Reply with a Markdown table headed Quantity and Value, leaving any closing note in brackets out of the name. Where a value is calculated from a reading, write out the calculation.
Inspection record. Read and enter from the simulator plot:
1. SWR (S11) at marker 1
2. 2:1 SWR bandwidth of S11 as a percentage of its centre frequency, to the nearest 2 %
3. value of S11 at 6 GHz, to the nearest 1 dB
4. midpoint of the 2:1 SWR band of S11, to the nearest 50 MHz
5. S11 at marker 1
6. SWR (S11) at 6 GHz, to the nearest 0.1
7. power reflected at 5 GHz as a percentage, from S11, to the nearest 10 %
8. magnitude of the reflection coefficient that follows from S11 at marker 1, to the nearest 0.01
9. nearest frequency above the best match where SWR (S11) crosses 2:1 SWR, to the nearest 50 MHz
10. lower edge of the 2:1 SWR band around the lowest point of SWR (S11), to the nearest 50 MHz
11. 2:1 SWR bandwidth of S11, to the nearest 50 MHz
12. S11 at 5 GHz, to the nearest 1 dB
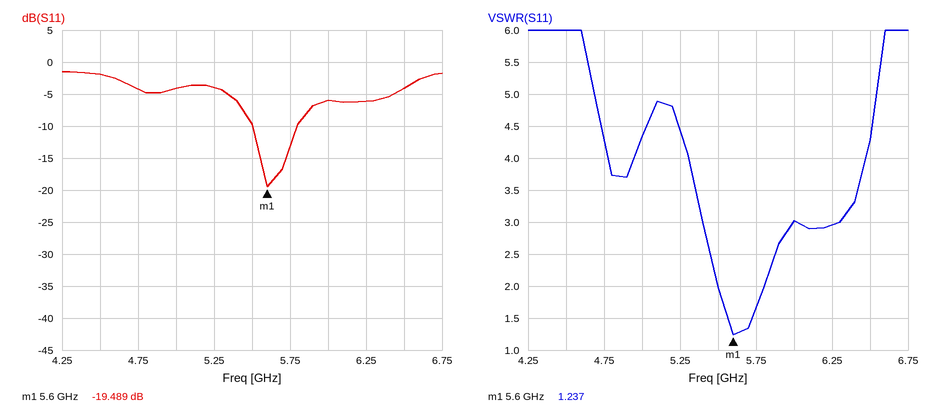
| Quantity | Value |
|---|---|
| SWR (S11) at marker 1 | 1.237 |
| 2:1 SWR bandwidth of S11 as a percentage of its centre frequency, to the nearest 2 % | 300 MHz / 5.65 GHz ≈ 5.31 %, so 6 % to the nearest 2 % |
| value of S11 at 6 GHz, to the nearest 1 dB | -6 dB |
| midpoint of the 2:1 SWR band of S11, to the nearest 50 MHz | 5.65 GHz |
| S11 at marker 1 | -19.489 dB |
| SWR (S11) at 6 GHz, to the nearest 0.1 | 3.0 |
| power reflected at 5 GHz as a percentage, from S11, to the nearest 10 % | 10^(-4/10) ≈ 40 % |
| magnitude of the reflection coefficient that follows from S11 at marker 1, to the nearest 0.01 | 10^(-19.489/20) ≈ 0.11 |
| nearest frequency above the best match where SWR (S11) crosses 2:1 SWR, to the nearest 50 MHz | 5.80 GHz |
| lower edge of the 2:1 SWR band around the lowest point of SWR (S11), to the nearest 50 MHz | 5.50 GHz |
| 2:1 SWR bandwidth of S11, to the nearest 50 MHz | 5.80 GHz − 5.50 GHz = 300 MHz |
| S11 at 5 GHz, to the nearest 1 dB | -4 dB |
